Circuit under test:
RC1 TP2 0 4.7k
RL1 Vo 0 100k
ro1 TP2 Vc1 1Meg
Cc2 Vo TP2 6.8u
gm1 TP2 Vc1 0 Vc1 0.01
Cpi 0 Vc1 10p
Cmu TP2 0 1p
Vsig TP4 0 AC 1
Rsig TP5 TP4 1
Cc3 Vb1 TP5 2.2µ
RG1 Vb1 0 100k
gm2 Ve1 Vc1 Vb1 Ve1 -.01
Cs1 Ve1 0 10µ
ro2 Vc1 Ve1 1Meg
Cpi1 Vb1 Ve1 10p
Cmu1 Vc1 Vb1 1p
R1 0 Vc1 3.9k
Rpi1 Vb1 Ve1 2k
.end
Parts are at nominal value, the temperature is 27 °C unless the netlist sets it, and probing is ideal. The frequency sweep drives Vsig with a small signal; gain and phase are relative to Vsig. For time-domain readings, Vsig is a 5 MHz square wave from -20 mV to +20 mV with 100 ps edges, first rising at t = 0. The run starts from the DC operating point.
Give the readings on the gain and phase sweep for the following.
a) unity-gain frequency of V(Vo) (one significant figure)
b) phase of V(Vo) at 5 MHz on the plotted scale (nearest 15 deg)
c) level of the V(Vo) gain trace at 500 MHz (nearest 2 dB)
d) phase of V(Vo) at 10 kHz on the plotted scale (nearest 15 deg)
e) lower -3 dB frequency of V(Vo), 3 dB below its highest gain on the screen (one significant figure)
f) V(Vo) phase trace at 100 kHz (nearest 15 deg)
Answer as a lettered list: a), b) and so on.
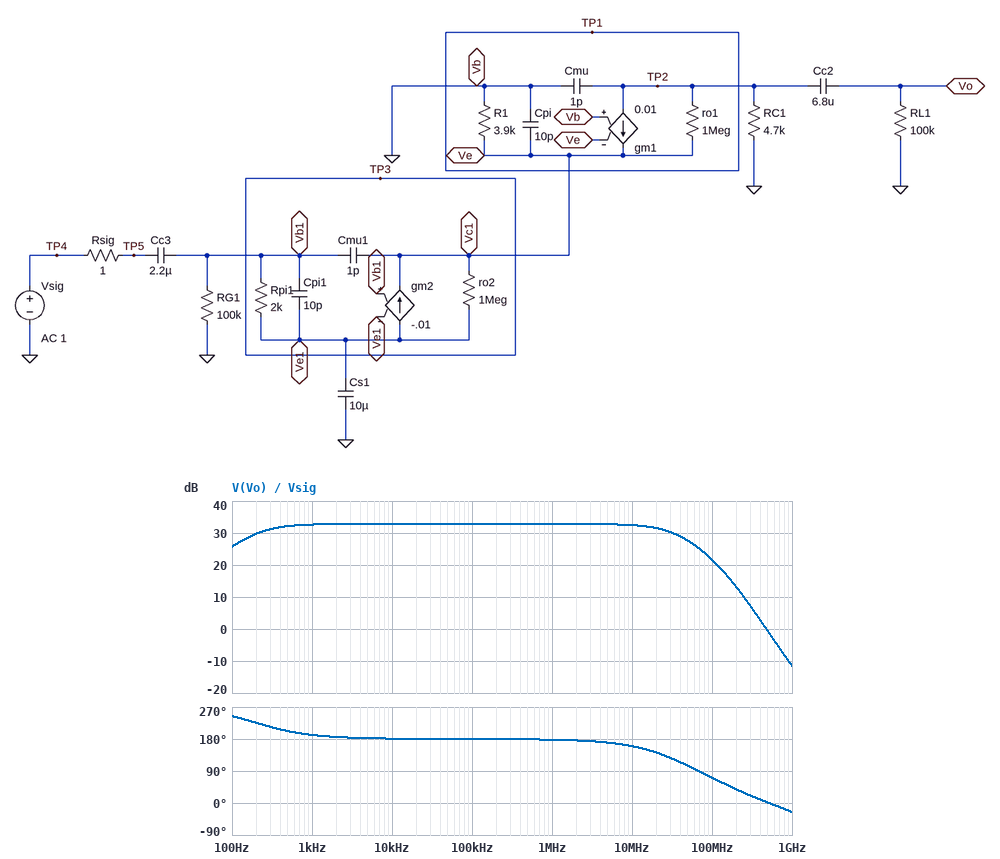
a) 500 MHz
b) 165 deg
c) 0 dB
d) 180 deg
e) 200 Hz
f) 180 deg
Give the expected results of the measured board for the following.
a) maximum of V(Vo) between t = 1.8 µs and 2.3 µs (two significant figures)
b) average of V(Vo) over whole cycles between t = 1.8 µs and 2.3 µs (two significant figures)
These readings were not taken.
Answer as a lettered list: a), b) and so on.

a) 4.0 mV
b) -870 mV
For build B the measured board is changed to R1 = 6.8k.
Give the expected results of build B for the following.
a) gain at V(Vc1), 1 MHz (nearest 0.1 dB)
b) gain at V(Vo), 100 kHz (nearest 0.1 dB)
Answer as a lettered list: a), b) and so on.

a) -0.1 dB
b) 32.9 dB
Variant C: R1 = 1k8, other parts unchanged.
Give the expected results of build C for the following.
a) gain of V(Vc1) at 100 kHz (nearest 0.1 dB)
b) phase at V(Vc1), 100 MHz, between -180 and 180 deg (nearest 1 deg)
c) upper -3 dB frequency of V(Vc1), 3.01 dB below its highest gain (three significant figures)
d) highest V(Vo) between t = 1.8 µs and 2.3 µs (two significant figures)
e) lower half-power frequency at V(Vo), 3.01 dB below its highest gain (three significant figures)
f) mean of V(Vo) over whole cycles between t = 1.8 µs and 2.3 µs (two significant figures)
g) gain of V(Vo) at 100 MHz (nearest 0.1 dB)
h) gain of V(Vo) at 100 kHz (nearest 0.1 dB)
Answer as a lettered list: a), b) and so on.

a) -0.4 dB
b) 143 deg
c) 153 MHz
d) 3.9 mV
e) 203 Hz
f) -850 mV
g) 21.5 dB
h) 32.6 dB
